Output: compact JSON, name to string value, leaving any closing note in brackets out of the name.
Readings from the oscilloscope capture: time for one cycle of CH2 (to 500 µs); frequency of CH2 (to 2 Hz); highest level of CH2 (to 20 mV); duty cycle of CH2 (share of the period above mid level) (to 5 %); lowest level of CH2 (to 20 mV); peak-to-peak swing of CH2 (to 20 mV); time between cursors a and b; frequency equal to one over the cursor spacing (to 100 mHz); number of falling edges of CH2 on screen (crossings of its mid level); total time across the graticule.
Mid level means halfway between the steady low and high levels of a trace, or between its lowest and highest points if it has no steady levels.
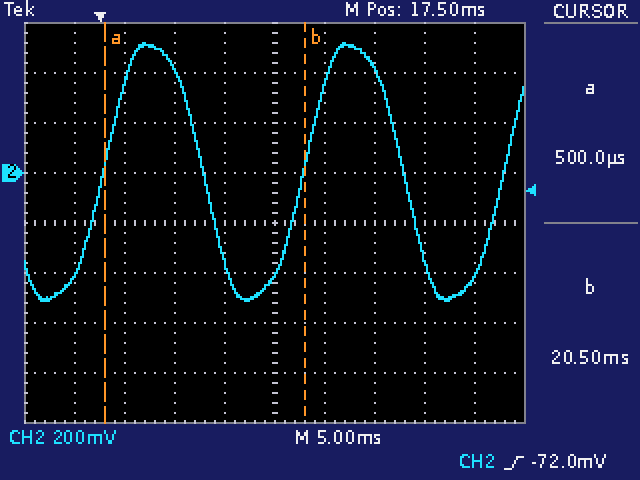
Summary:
{"time for one cycle of CH2": "20.0 ms", "frequency of CH2": "50 Hz", "highest level of CH2": "520 mV", "duty cycle of CH2 (share of the period above mid level)": "50 %", "lowest level of CH2": "-520 mV", "peak-to-peak swing of CH2": "1.04 V", "time between cursors a and b": "20.0 ms", "frequency equal to one over the cursor spacing": "50.0 Hz", "number of falling edges of CH2 on screen": "2", "total time across the graticule": "50 ms"}
